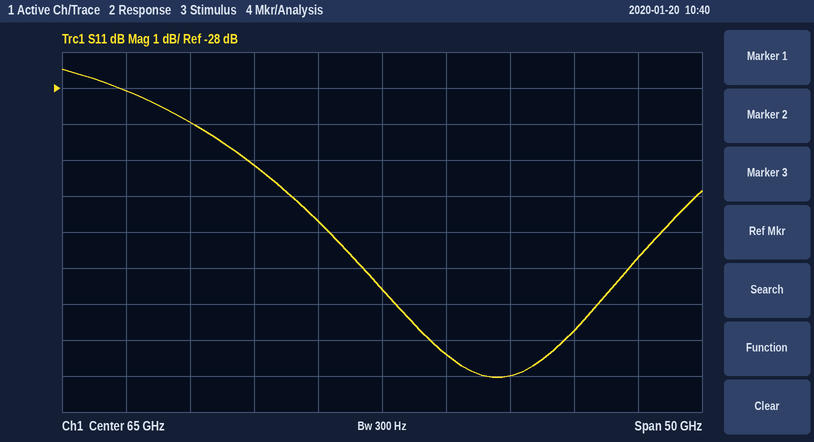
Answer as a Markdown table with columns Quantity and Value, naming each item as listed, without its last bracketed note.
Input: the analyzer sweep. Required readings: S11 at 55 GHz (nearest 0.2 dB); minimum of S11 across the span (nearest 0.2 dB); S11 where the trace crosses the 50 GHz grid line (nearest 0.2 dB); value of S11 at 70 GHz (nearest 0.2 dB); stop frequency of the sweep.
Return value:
| Quantity | Value |
|---|---|
| S11 at 55 GHz | -30.2 dB |
| minimum of S11 across the span | -36.0 dB |
| S11 where the trace crosses the 50 GHz grid line | -29.0 dB |
| value of S11 at 70 GHz | -35.4 dB |
| stop frequency of the sweep | 90 GHz |
